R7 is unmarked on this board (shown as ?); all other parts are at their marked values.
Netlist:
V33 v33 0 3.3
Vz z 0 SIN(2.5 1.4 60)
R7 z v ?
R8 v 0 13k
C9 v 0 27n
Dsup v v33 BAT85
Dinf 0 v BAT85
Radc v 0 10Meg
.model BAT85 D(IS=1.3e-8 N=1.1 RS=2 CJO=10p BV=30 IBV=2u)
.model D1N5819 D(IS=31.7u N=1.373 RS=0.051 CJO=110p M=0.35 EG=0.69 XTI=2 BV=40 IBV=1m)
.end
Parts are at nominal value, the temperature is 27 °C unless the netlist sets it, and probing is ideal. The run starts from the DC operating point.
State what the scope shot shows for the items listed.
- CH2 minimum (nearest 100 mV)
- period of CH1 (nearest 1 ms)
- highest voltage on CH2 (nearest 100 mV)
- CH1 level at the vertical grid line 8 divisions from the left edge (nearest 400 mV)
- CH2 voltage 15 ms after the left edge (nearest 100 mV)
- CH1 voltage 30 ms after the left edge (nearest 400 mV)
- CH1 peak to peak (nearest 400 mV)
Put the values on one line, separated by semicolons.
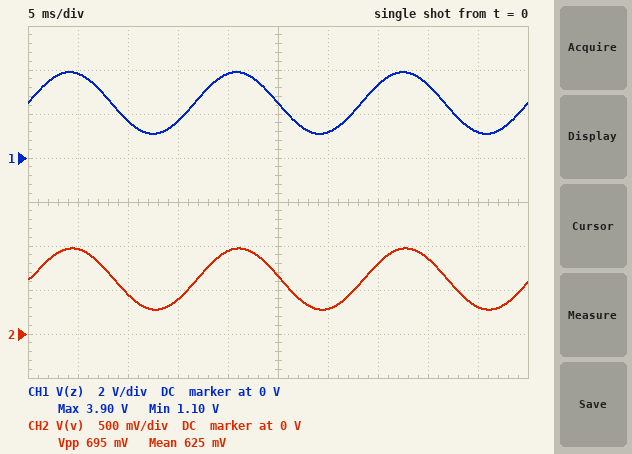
300 mV; 17 ms; 1.0 V; 3.2 V; 400 mV; 1.2 V; 2.8 V
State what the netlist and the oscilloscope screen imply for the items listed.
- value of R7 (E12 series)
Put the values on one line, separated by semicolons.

39 kΩ
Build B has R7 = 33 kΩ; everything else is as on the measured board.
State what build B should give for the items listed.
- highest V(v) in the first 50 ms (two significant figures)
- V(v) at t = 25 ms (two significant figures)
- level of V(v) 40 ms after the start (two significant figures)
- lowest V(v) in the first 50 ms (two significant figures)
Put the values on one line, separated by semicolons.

1.1 V; 740 mV; 970 mV; 310 mV
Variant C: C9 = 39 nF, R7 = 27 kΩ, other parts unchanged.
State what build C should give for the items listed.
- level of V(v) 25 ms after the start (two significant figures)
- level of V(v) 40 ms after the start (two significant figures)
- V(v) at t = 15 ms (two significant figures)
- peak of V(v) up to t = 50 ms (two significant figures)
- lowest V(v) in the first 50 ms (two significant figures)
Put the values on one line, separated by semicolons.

870 mV; 1.1 V; 500 mV; 1.3 V; 360 mV
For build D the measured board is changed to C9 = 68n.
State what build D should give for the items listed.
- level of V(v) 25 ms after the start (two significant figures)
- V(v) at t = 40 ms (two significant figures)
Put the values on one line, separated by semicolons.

710 mV; 880 mV
